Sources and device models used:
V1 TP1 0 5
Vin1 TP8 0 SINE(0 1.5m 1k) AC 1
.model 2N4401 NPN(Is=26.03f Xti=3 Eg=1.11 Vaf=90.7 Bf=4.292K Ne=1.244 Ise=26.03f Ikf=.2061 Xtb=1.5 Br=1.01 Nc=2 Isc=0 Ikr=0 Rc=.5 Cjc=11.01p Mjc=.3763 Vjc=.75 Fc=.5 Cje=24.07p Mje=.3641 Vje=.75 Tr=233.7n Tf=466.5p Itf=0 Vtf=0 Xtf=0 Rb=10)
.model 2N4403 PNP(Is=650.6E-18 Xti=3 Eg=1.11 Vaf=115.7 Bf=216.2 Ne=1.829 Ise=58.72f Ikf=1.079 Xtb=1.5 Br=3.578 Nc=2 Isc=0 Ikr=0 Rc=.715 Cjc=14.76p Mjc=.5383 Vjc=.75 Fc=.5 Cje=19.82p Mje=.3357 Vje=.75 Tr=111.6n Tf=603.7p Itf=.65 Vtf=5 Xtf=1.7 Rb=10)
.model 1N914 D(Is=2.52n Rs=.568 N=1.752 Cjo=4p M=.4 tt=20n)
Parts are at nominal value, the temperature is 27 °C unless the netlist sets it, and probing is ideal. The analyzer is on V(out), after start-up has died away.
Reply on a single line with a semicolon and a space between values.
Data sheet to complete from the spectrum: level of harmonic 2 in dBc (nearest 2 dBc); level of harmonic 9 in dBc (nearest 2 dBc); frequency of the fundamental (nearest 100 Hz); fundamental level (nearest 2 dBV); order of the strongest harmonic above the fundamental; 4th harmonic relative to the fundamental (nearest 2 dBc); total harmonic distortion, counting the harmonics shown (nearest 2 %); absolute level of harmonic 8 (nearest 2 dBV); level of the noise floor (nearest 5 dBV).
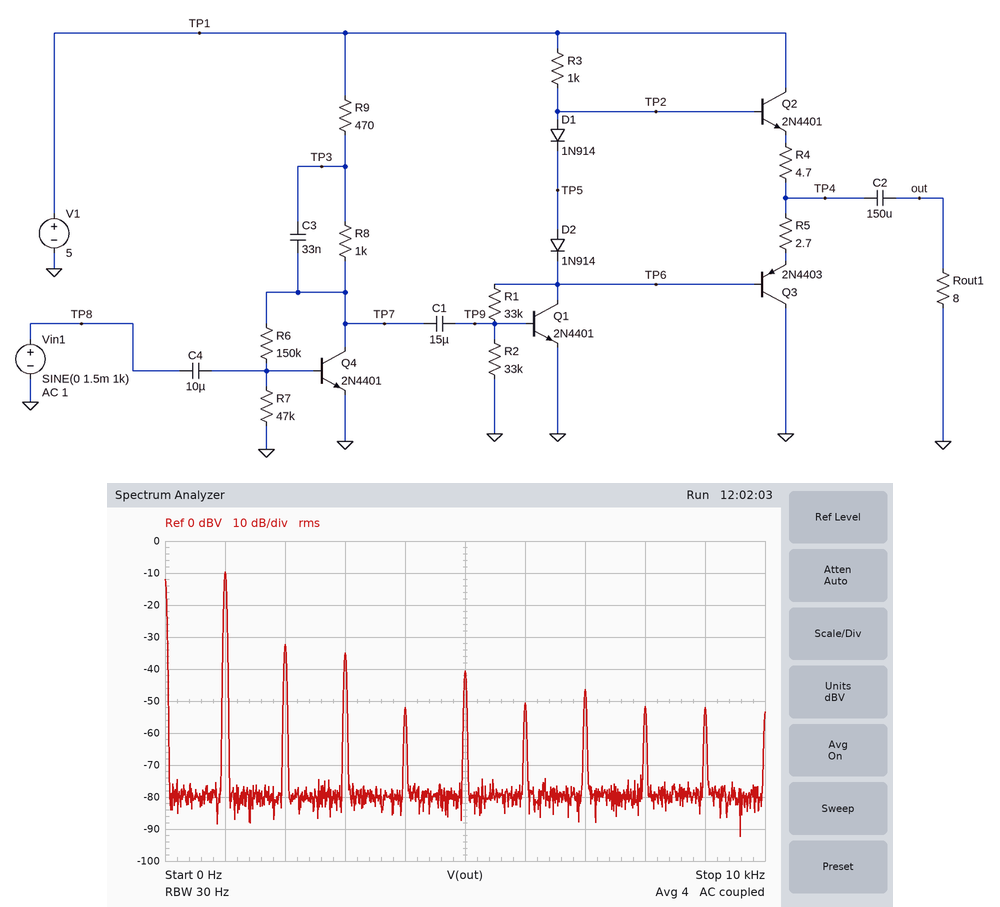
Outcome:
-22 dBc; -42 dBc; 1.0 kHz; -10 dBV; 2; -42 dBc; 10 %; -52 dBV; -80 dBV
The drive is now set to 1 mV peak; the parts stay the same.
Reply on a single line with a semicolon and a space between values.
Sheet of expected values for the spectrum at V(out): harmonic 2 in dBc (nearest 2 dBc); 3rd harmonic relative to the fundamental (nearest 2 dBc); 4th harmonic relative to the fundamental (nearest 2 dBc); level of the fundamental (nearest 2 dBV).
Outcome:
-24 dBc; -22 dBc; -40 dBc; -14 dBV
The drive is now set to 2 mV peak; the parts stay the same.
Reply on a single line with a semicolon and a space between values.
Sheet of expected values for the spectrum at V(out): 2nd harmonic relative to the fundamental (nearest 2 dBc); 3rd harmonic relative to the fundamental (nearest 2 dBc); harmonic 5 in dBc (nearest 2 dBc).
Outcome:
-20 dBc; -28 dBc; -32 dBc
